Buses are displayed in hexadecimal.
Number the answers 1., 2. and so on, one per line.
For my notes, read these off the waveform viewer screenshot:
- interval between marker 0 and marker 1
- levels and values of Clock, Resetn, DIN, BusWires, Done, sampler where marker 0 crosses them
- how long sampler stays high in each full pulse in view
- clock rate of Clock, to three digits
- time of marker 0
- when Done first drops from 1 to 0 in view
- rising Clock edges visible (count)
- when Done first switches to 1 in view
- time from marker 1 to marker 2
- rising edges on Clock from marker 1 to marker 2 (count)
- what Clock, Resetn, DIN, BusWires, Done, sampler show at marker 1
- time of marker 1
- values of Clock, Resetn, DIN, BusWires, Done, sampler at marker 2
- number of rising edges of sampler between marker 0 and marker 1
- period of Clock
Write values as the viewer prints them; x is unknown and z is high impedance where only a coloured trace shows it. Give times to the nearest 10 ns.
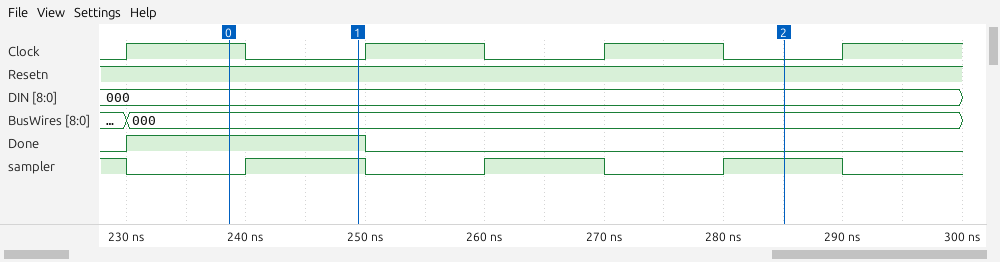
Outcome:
1. 10 ns
2. Clock=1, Resetn=1, DIN=000, BusWires=000, Done=1, sampler=0
3. 10 ns, 10 ns, 10 ns
4. 50.0 MHz
5. 240 ns
6. 250 ns
7. 4
8. 230 ns
9. 40 ns
10. 2
11. Clock=0, Resetn=1, DIN=000, BusWires=000, Done=1, sampler=1
12. 250 ns
13. Clock=0, Resetn=1, DIN=000, BusWires=000, Done=0, sampler=1
14. 1
15. 20 ns
